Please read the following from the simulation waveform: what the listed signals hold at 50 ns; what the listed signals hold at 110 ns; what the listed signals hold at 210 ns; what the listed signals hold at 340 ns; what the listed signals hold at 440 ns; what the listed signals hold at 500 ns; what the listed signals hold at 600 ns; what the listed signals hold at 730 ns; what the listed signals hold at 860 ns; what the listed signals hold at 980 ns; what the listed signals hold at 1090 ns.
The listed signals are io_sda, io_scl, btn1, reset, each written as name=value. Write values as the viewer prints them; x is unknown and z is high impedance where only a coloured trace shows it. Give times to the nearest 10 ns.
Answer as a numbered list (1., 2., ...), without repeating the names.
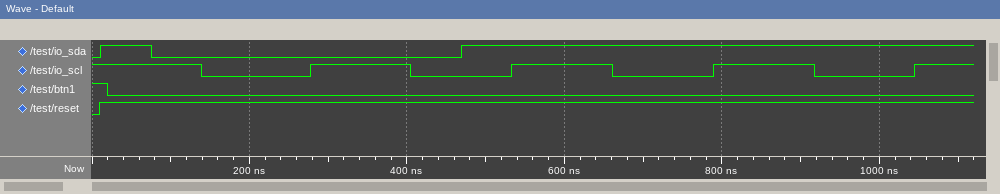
1. io_sda=1, io_scl=1, btn1=0, reset=1
2. io_sda=0, io_scl=1, btn1=0, reset=1
3. io_sda=0, io_scl=0, btn1=0, reset=1
4. io_sda=0, io_scl=1, btn1=0, reset=1
5. io_sda=0, io_scl=0, btn1=0, reset=1
6. io_sda=1, io_scl=0, btn1=0, reset=1
7. io_sda=1, io_scl=1, btn1=0, reset=1
8. io_sda=1, io_scl=0, btn1=0, reset=1
9. io_sda=1, io_scl=1, btn1=0, reset=1
10. io_sda=1, io_scl=0, btn1=0, reset=1
11. io_sda=1, io_scl=1, btn1=0, reset=1
